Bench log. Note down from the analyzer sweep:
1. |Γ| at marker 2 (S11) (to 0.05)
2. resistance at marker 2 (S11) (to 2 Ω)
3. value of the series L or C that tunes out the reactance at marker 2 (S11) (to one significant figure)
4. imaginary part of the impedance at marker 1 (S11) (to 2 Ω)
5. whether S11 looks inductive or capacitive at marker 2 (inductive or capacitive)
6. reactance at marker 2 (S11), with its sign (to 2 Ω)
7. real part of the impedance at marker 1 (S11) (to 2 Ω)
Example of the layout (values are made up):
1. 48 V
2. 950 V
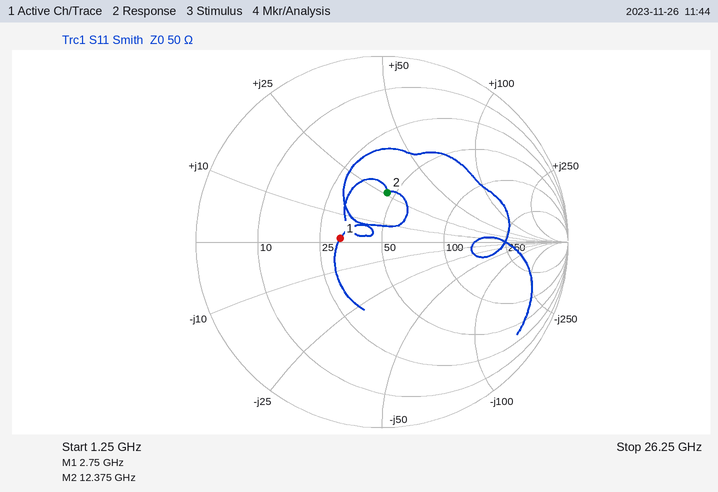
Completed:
1. 0.25
2. 46 Ω
3. 500 fF
4. +2 Ω
5. inductive
6. +26 Ω
7. 32 Ω
